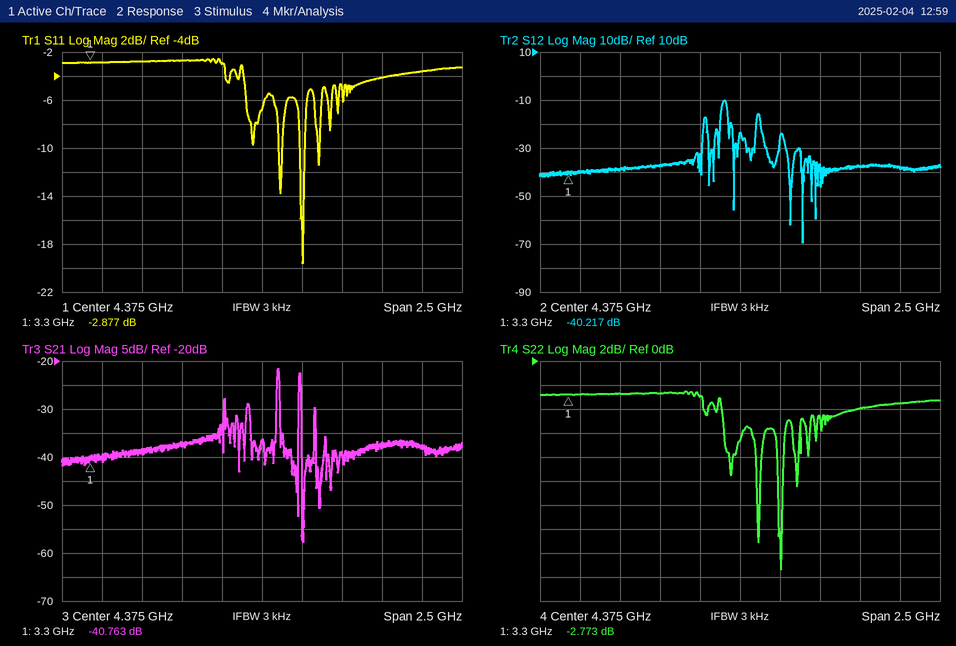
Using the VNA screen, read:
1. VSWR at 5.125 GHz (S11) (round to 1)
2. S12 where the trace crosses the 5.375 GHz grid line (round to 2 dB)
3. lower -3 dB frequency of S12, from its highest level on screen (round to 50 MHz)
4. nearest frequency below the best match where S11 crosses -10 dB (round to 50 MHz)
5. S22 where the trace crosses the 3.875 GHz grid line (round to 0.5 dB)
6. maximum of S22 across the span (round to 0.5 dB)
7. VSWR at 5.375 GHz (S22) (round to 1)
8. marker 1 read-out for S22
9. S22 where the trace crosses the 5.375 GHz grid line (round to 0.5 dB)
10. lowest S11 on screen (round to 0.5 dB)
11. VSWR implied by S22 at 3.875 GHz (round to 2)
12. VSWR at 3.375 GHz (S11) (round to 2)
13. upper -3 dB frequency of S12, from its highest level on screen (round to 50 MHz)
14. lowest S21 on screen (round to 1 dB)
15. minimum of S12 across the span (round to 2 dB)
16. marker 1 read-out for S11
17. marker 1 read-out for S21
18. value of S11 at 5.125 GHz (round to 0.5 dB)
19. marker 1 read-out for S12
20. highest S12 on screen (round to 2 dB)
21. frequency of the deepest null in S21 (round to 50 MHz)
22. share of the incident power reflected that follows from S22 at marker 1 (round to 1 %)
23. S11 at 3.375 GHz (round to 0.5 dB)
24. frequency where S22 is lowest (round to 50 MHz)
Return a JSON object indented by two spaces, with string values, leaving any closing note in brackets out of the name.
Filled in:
{
  "VSWR at 5.125 GHz (S11)": "4",
  "S12 where the trace crosses the 5.375 GHz grid line": "-38 dB",
  "lower -3 dB frequency of S12, from its highest level on screen": "4.25 GHz",
  "nearest frequency below the best match where S11 crosses -10 dB": "4.60 GHz",
  "S22 where the trace crosses the 3.875 GHz grid line": "-2.5 dB",
  "maximum of S22 across the span": "-2.5 dB",
  "VSWR at 5.375 GHz (S22)": "5",
  "marker 1 read-out for S22": "-2.773 dB",
  "S22 where the trace crosses the 5.375 GHz grid line": "-3.5 dB",
  "lowest S11 on screen": "-19.5 dB",
  "VSWR implied by S22 at 3.875 GHz": "6",
  "VSWR at 3.375 GHz (S11)": "6",
  "upper -3 dB frequency of S12, from its highest level on screen": "4.30 GHz",
  "lowest S21 on screen": "-58 dB",
  "minimum of S12 across the span": "-70 dB",
  "marker 1 read-out for S11": "-2.877 dB",
  "marker 1 read-out for S21": "-40.763 dB",
  "value of S11 at 5.125 GHz": "-4.0 dB",
  "marker 1 read-out for S12": "-40.217 dB",
  "highest S12 on screen": "-10 dB",
  "frequency of the deepest null in S21": "4.65 GHz",
  "share of the incident power reflected that follows from S22 at marker 1": "53 %",
  "S11 at 3.375 GHz": "-3.0 dB",
  "frequency where S22 is lowest": "4.65 GHz"
}
